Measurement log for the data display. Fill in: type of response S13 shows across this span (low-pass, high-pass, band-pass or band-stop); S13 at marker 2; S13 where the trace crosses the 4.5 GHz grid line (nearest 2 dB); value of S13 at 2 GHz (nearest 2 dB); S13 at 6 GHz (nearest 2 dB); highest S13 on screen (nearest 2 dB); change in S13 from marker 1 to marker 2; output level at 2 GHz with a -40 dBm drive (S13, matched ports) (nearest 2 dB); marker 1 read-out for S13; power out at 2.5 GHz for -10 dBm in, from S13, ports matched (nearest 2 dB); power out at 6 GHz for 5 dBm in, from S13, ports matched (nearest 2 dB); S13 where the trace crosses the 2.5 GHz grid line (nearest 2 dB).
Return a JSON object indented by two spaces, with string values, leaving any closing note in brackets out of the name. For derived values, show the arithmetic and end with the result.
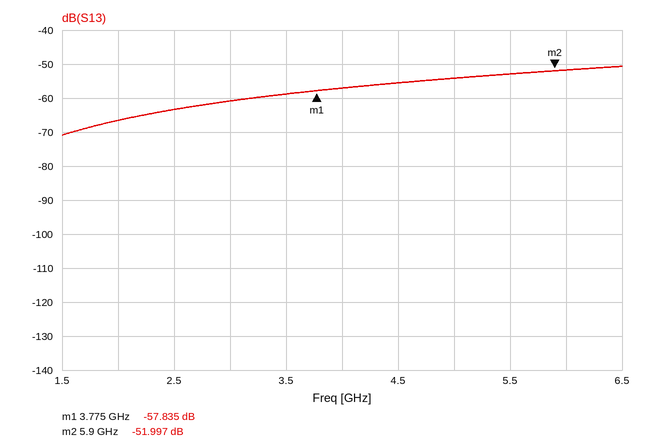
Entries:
{
  "type of response S13 shows across this span": "high-pass",
  "S13 at marker 2": "-51.997 dB",
  "S13 where the trace crosses the 4.5 GHz grid line": "-56 dB",
  "value of S13 at 2 GHz": "-66 dB",
  "S13 at 6 GHz": "-52 dB",
  "highest S13 on screen": "-50 dB",
  "change in S13 from marker 1 to marker 2": "-51.997 − (-57.835) = 5.838 dB",
  "output level at 2 GHz with a -40 dBm drive (S13, matched ports)": "-40 dBm + (-66 dB) = -106 dBm",
  "marker 1 read-out for S13": "-57.835 dB",
  "power out at 2.5 GHz for -10 dBm in, from S13, ports matched": "-10 dBm + (-64 dB) = -74 dBm",
  "power out at 6 GHz for 5 dBm in, from S13, ports matched": "5 dBm + (-52 dB) = -46 dBm",
  "S13 where the trace crosses the 2.5 GHz grid line": "-64 dB"
}
